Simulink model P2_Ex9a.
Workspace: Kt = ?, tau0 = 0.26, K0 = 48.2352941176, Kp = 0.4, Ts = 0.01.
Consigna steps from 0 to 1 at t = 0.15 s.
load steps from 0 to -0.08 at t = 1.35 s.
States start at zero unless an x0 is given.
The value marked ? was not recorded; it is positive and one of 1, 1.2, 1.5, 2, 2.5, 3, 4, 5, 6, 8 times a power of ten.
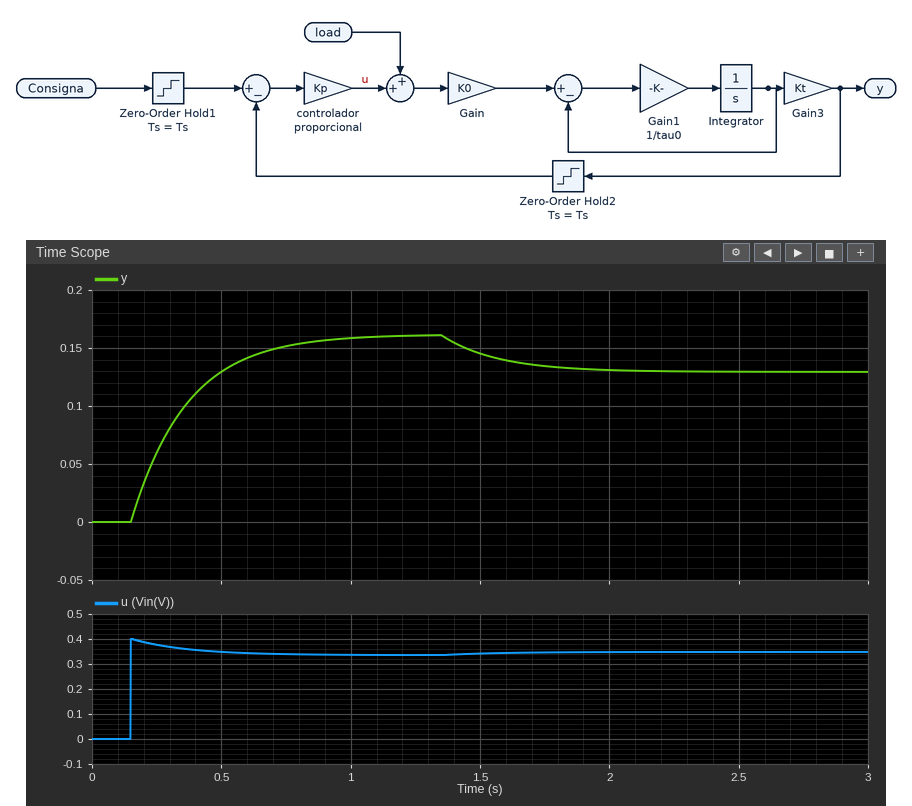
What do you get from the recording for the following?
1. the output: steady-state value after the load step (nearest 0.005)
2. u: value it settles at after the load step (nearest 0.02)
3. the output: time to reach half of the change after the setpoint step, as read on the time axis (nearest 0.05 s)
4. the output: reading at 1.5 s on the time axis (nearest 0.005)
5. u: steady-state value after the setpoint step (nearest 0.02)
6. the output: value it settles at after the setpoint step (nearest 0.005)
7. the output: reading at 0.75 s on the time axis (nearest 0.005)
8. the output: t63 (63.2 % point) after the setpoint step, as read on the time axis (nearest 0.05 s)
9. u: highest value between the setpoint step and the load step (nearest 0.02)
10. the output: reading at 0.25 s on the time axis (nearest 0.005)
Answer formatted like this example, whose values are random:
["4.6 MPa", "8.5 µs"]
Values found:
["0.130", "0.34", "0.30 s", "0.145", "0.34", "0.160", "0.150", "0.35 s", "0.40", "0.060"]
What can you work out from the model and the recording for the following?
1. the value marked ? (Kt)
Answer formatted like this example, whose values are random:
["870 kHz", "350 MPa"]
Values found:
["0.01"]
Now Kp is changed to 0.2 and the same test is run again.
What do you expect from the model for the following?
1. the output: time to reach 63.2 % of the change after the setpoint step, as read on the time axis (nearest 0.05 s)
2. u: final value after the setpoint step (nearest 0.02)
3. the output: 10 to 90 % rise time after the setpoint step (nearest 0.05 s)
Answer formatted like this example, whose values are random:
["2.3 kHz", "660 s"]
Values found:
["0.40 s", "0.18", "0.50 s"]
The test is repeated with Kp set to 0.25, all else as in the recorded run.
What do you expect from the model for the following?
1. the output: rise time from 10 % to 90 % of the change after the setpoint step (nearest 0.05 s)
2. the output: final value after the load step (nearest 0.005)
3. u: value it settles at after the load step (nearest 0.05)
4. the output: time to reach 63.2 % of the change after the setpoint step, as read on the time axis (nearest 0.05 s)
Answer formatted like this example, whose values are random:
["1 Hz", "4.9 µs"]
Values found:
["0.50 s", "0.075", "0.25", "0.40 s"]
